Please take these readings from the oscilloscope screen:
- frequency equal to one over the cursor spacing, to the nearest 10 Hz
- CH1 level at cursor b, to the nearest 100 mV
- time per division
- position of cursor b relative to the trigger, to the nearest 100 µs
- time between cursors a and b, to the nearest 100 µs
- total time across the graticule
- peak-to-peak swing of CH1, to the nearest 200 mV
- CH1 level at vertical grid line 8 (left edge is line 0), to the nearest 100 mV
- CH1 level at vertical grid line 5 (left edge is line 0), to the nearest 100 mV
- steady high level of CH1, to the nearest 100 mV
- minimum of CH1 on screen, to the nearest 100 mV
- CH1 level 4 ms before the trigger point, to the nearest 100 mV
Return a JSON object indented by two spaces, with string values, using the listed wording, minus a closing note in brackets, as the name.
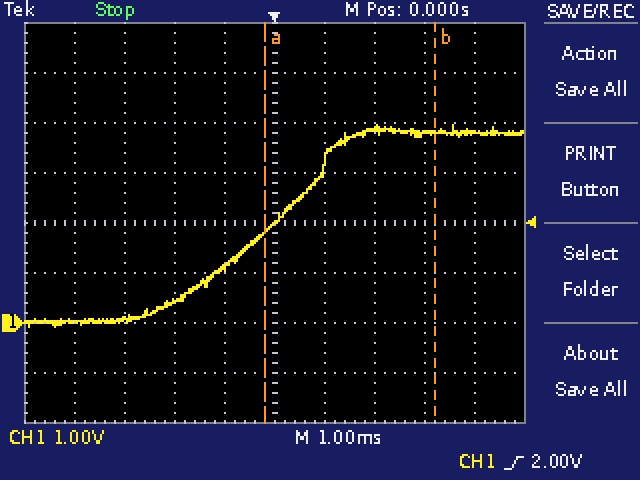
{
  "frequency equal to one over the cursor spacing, to the nearest 10 Hz": "290 Hz",
  "CH1 level at cursor b, to the nearest 100 mV": "3.8 V",
  "time per division": "1 ms",
  "position of cursor b relative to the trigger, to the nearest 100 µs": "+3.2 ms",
  "time between cursors a and b, to the nearest 100 µs": "3.4 ms",
  "total time across the graticule": "10 ms",
  "peak-to-peak swing of CH1, to the nearest 200 mV": "4.0 V",
  "CH1 level at vertical grid line 8 (left edge is line 0), to the nearest 100 mV": "3.8 V",
  "CH1 level at vertical grid line 5 (left edge is line 0), to the nearest 100 mV": "2.0 V",
  "steady high level of CH1, to the nearest 100 mV": "3.8 V",
  "minimum of CH1 on screen, to the nearest 100 mV": "-100 mV",
  "CH1 level 4 ms before the trigger point, to the nearest 100 mV": "0.0 V"
}
